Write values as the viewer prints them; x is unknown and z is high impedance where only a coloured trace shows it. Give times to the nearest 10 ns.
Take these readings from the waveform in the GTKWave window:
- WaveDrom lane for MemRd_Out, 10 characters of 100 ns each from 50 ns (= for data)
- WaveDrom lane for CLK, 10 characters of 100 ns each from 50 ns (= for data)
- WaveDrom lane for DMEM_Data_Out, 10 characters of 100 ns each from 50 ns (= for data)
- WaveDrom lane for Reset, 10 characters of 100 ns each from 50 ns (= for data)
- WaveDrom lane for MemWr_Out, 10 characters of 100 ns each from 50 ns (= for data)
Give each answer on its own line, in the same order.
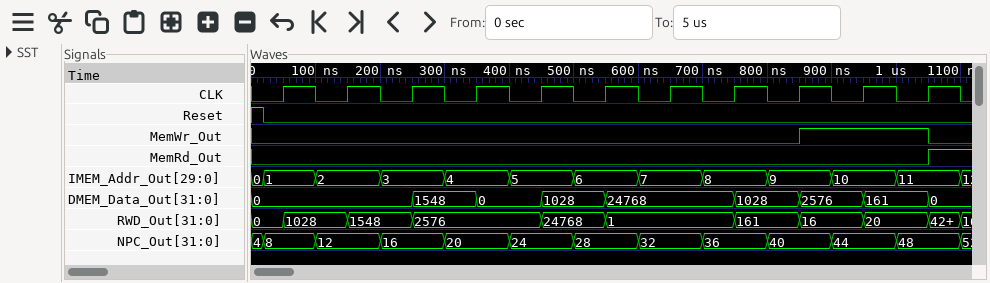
{name: 'MemRd_Out', wave: '0.........'}
{name: 'CLK', wave: 'p.........'}
{name: 'DMEM_Data_Out', wave: '=.====.===', data: '0 1548 0 1028 24768 1028 2576 161'}
{name: 'Reset', wave: '0.........'}
{name: 'MemWr_Out', wave: '0.......1.'}
